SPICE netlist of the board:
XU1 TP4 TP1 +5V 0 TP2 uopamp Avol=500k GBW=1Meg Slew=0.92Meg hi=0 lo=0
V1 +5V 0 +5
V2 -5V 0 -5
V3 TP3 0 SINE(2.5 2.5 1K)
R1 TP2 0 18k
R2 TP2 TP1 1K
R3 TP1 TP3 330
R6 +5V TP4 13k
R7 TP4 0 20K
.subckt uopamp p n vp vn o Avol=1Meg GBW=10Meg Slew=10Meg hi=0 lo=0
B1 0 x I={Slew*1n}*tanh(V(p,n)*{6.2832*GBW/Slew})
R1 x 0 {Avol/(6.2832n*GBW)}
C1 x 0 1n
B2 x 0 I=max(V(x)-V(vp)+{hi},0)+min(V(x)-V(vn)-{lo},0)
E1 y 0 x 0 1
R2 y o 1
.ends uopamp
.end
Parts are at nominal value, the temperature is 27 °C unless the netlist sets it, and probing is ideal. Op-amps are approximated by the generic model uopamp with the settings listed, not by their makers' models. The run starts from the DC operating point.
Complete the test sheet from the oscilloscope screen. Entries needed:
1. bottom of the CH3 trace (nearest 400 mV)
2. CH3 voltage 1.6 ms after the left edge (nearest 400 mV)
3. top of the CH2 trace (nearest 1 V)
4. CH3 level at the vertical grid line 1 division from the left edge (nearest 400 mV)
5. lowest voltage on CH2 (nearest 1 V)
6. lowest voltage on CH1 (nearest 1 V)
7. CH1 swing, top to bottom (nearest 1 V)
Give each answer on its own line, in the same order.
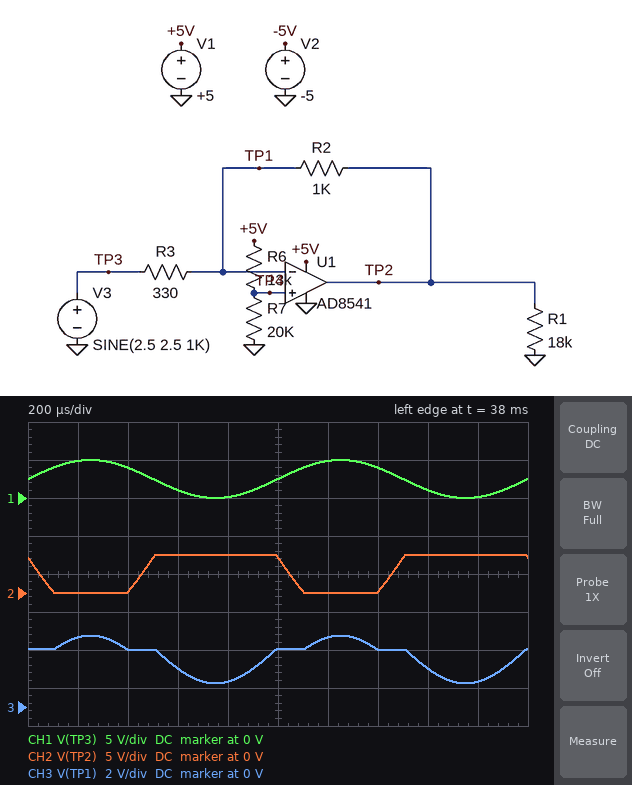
1.2 V
2.0 V
5 V
3.6 V
0 V
0 V
5 V
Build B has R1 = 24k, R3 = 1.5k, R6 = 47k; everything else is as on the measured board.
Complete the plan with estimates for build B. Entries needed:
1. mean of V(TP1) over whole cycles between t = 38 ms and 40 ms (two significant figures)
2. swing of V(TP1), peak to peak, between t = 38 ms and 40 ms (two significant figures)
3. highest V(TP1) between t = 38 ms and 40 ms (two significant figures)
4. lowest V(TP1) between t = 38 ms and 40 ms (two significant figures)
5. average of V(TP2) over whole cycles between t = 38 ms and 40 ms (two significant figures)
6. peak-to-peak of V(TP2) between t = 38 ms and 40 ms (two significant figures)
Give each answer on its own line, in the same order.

1.6 V
510 mV
2.0 V
1.5 V
1.0 V
2.5 V
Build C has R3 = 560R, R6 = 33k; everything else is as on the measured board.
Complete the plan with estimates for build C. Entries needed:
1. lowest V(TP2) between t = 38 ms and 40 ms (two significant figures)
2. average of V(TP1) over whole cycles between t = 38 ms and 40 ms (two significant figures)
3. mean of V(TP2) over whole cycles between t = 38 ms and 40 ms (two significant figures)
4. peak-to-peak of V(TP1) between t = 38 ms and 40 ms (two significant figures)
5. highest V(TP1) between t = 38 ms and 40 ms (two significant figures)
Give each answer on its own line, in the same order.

1.3 mV
2.3 V
1.8 V
1.4 V
3.2 V
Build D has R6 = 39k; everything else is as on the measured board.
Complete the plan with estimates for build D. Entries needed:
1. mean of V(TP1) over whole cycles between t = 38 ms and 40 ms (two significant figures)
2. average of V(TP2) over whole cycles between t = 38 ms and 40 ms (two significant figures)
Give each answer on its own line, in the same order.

2.3 V
1.8 V
